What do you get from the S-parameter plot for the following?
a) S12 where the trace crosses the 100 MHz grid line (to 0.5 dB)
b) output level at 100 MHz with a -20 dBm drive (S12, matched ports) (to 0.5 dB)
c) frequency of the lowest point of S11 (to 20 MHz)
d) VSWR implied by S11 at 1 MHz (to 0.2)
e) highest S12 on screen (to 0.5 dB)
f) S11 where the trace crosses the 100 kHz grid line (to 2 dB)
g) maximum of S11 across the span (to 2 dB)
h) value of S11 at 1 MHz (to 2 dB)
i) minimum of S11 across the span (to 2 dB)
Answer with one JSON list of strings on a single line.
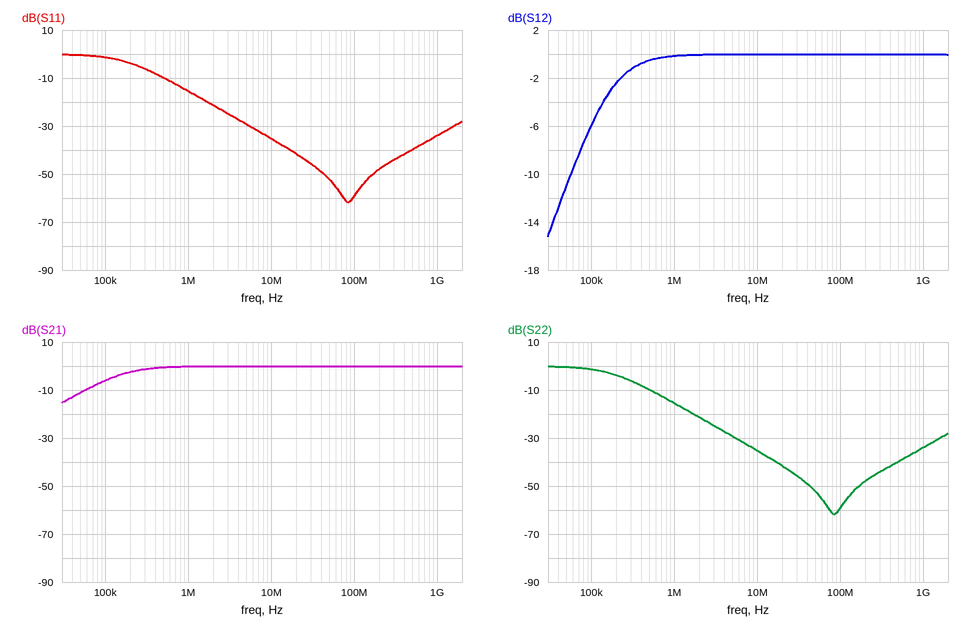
["0.0 dB", "-20.0 dBm", "80 MHz", "1.4", "0.0 dB", "-2 dB", "0 dB", "-16 dB", "-62 dB"]
